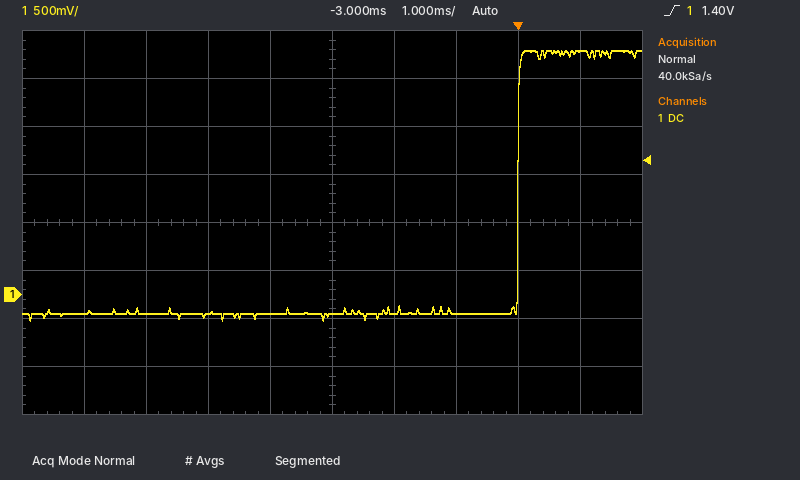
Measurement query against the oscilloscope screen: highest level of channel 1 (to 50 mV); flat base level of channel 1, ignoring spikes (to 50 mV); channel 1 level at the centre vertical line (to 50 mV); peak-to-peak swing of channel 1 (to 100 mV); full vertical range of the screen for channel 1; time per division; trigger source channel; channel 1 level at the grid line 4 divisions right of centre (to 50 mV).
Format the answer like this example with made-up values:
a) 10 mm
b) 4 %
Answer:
a) 2.55 V
b) -200 mV
c) -200 mV
d) 2.80 V
e) 4 V
f) 1 ms
g) channel 1
h) 2.55 V
